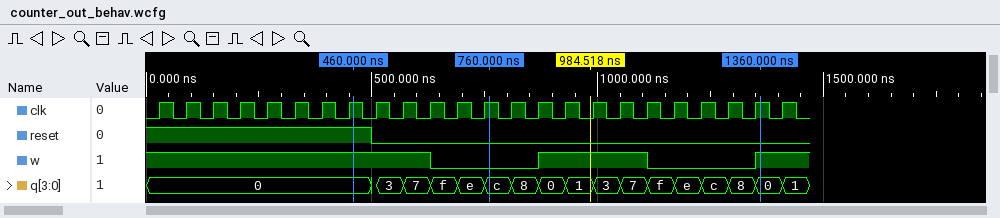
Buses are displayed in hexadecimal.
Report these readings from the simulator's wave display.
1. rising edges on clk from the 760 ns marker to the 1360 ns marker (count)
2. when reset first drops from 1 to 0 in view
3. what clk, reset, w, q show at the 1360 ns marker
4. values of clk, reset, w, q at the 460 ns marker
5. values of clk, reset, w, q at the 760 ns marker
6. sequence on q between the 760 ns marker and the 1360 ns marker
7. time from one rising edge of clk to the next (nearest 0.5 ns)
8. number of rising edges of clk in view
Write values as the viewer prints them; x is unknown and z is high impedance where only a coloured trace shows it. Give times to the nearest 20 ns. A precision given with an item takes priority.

10
500 ns
clk=1, reset=0, w=1, q=0
clk=1, reset=1, w=1, q=0
clk=1, reset=0, w=0, q=c
c, 8, 0, 1, 3, 7, f, e, c, 8, 0
60 ns
24
